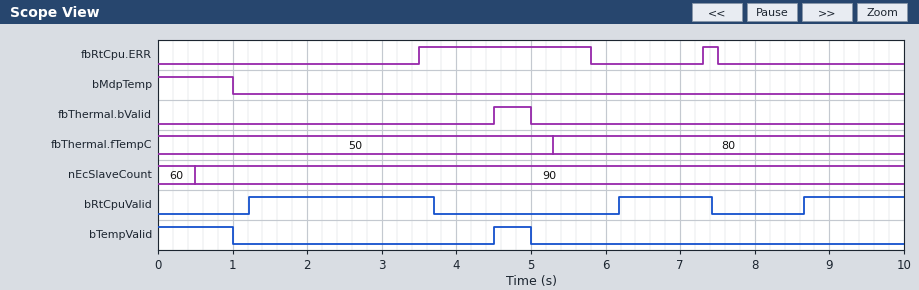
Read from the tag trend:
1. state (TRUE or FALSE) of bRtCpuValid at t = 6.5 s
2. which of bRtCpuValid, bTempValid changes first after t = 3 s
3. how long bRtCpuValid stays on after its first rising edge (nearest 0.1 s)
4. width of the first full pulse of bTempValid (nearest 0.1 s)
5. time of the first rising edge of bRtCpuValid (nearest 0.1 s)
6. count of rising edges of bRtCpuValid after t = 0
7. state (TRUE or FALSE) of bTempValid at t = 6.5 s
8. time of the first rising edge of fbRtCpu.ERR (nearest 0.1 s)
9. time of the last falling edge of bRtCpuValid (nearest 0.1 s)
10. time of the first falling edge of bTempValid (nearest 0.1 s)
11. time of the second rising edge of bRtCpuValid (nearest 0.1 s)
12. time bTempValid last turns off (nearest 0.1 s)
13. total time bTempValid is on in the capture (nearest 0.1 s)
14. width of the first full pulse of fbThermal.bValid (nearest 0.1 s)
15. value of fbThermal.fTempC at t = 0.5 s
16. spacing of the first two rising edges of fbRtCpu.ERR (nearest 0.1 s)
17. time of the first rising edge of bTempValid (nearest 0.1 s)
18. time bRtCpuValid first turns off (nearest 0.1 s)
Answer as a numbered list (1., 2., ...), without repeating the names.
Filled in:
1. TRUE
2. bRtCpuValid
3. 2.5 s
4. 0.5 s
5. 1.2 s
6. 3
7. FALSE
8. 3.5 s
9. 7.4 s
10. 1.0 s
11. 6.2 s
12. 5.0 s
13. 1.5 s
14. 0.5 s
15. 50
16. 3.8 s
17. 4.5 s
18. 3.7 s
